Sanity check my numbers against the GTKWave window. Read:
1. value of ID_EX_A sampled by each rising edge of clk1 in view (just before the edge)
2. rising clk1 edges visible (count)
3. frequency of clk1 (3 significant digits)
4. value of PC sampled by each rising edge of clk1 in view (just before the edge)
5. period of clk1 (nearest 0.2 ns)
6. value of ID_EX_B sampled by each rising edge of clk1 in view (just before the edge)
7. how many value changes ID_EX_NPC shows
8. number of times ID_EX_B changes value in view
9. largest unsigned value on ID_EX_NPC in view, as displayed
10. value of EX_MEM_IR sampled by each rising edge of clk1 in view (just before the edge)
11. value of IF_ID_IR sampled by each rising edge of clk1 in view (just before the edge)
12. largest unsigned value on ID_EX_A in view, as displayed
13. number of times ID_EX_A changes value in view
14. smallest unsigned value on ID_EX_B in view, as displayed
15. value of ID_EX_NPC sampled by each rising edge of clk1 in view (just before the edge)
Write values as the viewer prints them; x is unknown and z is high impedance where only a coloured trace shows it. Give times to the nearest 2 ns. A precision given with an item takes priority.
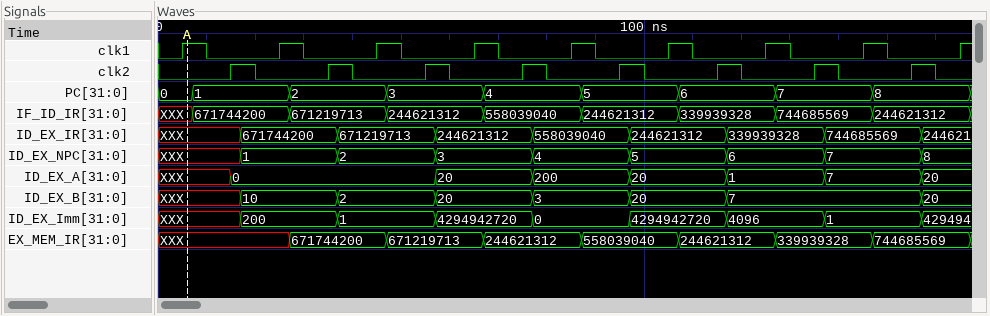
XXX, 0, 0, 20, 200, 20, 1, 7, 20
9
50.0 MHz
0, 1, 2, 3, 4, 5, 6, 7, 8
20 ns
XXX, 10, 2, 20, 3, 20, 7, 7, 20
8
7
8
XXX, XXX, 671744200, 671219713, 244621312, 558039040, 244621312, 339939328, 744685569
XXX, 671744200, 671219713, 244621312, 558039040, 244621312, 339939328, 744685569, 244621312
200
7
2
XXX, 1, 2, 3, 4, 5, 6, 7, 8
